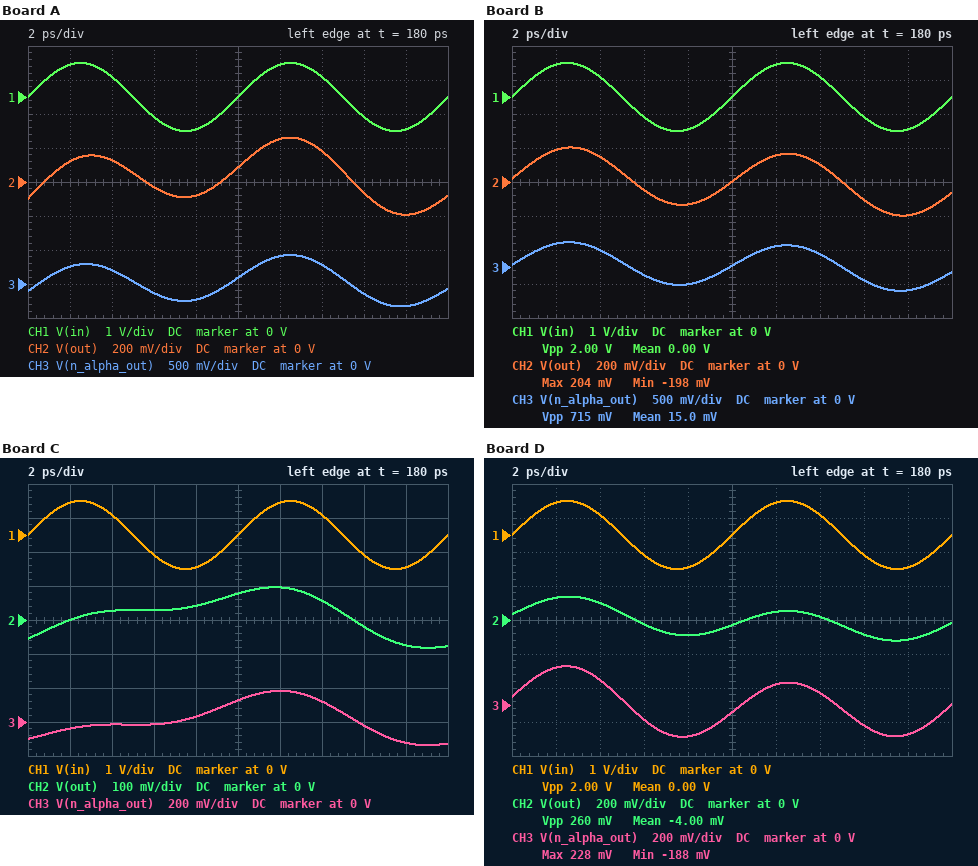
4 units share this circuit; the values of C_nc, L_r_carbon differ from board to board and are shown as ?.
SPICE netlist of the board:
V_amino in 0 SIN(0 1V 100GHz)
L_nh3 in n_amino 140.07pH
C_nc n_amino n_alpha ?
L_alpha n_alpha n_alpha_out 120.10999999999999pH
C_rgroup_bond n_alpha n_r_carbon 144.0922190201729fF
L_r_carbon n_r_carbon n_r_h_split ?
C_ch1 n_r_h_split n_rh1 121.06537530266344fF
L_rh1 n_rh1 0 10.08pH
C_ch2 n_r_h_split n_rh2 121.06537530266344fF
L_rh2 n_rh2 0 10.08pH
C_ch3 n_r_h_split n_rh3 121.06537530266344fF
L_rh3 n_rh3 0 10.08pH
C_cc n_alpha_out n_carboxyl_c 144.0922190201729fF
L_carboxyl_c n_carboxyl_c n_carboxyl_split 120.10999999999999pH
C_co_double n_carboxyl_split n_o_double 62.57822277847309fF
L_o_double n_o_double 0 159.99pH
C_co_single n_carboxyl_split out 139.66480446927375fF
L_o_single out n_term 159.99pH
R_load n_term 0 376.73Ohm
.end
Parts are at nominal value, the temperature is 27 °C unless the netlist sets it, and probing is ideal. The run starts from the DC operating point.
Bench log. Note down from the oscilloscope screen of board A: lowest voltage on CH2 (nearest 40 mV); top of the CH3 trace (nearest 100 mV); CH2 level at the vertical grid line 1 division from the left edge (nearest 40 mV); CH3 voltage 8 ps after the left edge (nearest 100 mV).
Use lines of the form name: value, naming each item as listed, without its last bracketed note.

lowest voltage on CH2: -200 mV
top of the CH3 trace: 400 mV
CH2 level at the vertical grid line 1 division from the left edge: 120 mV
CH3 voltage 8 ps after the left edge: -200 mV
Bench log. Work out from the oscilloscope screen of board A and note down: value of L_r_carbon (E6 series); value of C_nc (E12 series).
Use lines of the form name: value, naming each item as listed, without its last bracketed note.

value of L_r_carbon: 220 pH
value of C_nc: 120 fF
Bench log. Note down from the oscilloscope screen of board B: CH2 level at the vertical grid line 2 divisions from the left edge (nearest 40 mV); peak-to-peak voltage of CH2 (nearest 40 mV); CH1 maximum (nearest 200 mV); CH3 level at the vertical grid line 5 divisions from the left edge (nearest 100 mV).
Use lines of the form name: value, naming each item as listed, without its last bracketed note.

CH2 level at the vertical grid line 2 divisions from the left edge: 160 mV
peak-to-peak voltage of CH2: 400 mV
CH1 maximum: 1.0 V
CH3 level at the vertical grid line 5 divisions from the left edge: 0 V
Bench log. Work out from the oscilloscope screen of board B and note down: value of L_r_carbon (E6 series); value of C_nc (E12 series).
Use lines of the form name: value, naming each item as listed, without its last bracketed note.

value of L_r_carbon: 220 pH
value of C_nc: 390 fF
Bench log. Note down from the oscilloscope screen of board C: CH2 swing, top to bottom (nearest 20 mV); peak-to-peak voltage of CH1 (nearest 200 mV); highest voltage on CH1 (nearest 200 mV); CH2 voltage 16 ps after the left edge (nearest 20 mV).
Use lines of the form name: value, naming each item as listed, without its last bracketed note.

CH2 swing, top to bottom: 180 mV
peak-to-peak voltage of CH1: 2.0 V
highest voltage on CH1: 1.0 V
CH2 voltage 16 ps after the left edge: -20 mV
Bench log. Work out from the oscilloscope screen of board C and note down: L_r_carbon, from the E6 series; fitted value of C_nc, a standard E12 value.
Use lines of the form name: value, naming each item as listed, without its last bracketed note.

L_r_carbon, from the E6 series: 33 pH
fitted value of C_nc, a standard E12 value: 120 fF
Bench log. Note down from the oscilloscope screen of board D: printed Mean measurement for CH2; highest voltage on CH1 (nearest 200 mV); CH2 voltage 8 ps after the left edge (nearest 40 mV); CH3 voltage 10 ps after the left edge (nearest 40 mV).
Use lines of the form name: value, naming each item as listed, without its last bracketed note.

printed Mean measurement for CH2: -4.00 mV
highest voltage on CH1: 1.0 V
CH2 voltage 8 ps after the left edge: -80 mV
CH3 voltage 10 ps after the left edge: -40 mV
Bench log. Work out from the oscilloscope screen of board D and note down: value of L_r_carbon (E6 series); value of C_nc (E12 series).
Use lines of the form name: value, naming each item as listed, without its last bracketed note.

value of L_r_carbon: 68 pH
value of C_nc: 82 fF
